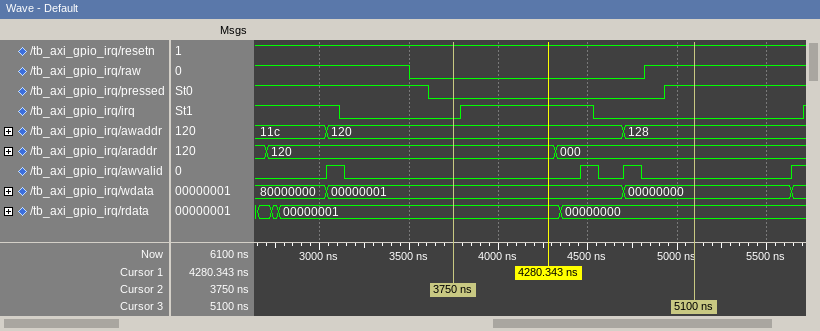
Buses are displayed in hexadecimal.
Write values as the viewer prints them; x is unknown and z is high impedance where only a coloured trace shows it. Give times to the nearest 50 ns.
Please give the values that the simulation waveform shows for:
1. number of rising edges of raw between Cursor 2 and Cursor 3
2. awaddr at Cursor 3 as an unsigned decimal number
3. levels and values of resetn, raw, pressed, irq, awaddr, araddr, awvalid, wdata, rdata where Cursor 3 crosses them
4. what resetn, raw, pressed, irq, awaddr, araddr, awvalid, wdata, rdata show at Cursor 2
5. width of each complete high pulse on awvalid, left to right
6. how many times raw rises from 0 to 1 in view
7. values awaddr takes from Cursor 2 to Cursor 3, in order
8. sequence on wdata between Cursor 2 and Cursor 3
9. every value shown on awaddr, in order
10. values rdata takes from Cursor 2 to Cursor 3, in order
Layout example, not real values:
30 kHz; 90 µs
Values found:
1; 296; resetn=1, raw=1, pressed=1, irq=0, awaddr=128, araddr=000, awvalid=0, wdata=00000000, rdata=00000000; resetn=1, raw=0, pressed=0, irq=0, awaddr=120, araddr=120, awvalid=0, wdata=00000001, rdata=00000001; 100 ns, 100 ns, 100 ns; 1; 120, 128; 00000001, 00000000; 11c, 120, 128; 00000001, 00000000
